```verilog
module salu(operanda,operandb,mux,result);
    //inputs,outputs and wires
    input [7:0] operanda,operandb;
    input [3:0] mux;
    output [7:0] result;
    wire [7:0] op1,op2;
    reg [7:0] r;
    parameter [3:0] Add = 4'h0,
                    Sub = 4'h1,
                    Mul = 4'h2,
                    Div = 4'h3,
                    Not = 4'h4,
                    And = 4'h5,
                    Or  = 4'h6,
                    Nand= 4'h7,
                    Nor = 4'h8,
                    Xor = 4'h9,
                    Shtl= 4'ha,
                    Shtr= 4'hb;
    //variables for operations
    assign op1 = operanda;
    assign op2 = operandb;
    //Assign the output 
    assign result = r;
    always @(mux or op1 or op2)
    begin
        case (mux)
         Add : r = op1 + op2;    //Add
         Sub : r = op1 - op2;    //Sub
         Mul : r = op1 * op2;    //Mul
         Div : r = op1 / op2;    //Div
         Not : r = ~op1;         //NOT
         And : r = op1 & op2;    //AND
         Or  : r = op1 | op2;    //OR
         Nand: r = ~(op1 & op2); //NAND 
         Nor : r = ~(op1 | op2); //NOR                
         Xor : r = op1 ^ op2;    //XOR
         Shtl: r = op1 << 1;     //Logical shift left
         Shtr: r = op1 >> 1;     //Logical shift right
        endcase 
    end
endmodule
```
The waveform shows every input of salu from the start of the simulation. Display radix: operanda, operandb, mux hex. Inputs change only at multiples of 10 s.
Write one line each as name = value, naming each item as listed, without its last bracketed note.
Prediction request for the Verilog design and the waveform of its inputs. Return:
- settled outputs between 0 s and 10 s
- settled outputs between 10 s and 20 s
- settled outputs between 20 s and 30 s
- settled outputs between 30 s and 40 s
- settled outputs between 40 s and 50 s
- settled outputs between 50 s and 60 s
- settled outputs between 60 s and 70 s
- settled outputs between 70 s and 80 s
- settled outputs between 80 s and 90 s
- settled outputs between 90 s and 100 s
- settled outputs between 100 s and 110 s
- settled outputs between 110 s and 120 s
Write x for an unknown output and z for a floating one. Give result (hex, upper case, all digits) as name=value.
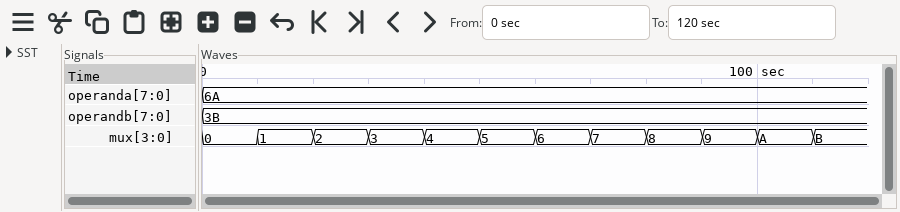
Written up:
settled outputs between 0 s and 10 s = result=A5
settled outputs between 10 s and 20 s = result=2F
settled outputs between 20 s and 30 s = result=6E
settled outputs between 30 s and 40 s = result=01
settled outputs between 40 s and 50 s = result=95
settled outputs between 50 s and 60 s = result=2A
settled outputs between 60 s and 70 s = result=7B
settled outputs between 70 s and 80 s = result=D5
settled outputs between 80 s and 90 s = result=84
settled outputs between 90 s and 100 s = result=51
settled outputs between 100 s and 110 s = result=D4
settled outputs between 110 s and 120 s = result=35
